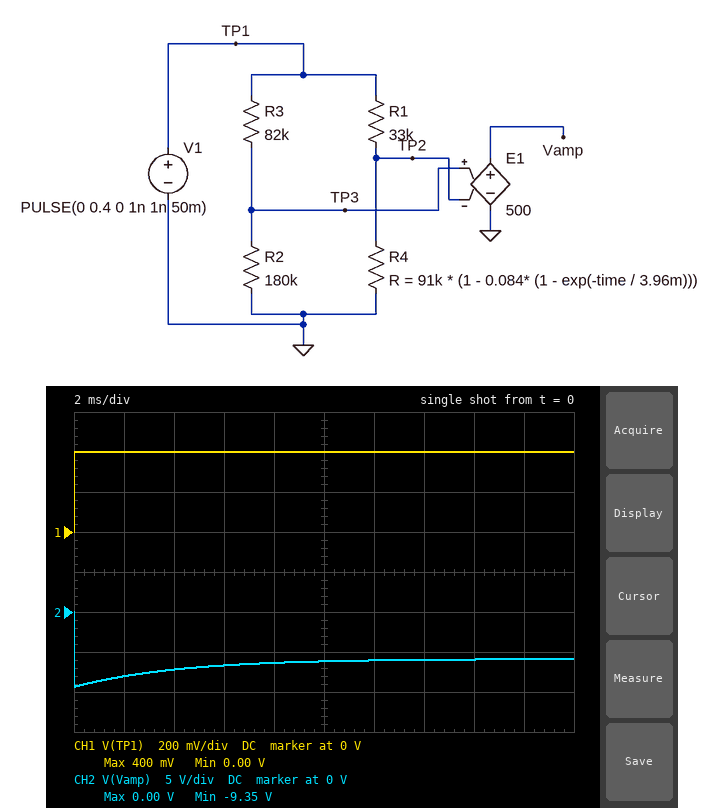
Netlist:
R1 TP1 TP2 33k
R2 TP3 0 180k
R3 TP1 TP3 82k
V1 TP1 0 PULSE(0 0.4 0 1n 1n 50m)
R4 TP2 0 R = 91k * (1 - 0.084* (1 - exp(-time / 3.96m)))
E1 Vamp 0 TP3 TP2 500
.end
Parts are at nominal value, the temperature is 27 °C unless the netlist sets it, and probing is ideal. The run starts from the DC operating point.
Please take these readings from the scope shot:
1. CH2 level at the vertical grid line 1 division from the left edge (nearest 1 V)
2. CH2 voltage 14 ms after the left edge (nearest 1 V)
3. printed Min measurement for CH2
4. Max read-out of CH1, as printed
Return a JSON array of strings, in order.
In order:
["-8 V", "-6 V", "-9.35 V", "400 mV"]
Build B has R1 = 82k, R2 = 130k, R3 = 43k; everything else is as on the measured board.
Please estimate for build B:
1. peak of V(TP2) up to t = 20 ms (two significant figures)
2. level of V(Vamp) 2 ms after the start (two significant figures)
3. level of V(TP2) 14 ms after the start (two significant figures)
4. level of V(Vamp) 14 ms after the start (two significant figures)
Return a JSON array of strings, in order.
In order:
["210 mV", "47 V", "200 mV", "49 V"]
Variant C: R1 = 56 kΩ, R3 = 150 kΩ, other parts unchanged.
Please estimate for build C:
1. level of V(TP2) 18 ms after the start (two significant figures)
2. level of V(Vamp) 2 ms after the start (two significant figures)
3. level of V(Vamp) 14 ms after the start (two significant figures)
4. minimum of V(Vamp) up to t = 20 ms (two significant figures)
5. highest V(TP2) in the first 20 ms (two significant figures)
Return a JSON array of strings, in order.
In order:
["240 mV", "-13 V", "-11 V", "-15 V", "250 mV"]
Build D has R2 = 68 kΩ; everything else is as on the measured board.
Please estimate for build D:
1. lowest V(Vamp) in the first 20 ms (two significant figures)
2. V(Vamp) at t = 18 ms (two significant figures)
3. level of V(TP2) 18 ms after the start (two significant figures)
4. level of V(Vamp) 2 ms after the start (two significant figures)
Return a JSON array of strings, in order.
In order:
["-56 V", "-53 V", "290 mV", "-55 V"]
